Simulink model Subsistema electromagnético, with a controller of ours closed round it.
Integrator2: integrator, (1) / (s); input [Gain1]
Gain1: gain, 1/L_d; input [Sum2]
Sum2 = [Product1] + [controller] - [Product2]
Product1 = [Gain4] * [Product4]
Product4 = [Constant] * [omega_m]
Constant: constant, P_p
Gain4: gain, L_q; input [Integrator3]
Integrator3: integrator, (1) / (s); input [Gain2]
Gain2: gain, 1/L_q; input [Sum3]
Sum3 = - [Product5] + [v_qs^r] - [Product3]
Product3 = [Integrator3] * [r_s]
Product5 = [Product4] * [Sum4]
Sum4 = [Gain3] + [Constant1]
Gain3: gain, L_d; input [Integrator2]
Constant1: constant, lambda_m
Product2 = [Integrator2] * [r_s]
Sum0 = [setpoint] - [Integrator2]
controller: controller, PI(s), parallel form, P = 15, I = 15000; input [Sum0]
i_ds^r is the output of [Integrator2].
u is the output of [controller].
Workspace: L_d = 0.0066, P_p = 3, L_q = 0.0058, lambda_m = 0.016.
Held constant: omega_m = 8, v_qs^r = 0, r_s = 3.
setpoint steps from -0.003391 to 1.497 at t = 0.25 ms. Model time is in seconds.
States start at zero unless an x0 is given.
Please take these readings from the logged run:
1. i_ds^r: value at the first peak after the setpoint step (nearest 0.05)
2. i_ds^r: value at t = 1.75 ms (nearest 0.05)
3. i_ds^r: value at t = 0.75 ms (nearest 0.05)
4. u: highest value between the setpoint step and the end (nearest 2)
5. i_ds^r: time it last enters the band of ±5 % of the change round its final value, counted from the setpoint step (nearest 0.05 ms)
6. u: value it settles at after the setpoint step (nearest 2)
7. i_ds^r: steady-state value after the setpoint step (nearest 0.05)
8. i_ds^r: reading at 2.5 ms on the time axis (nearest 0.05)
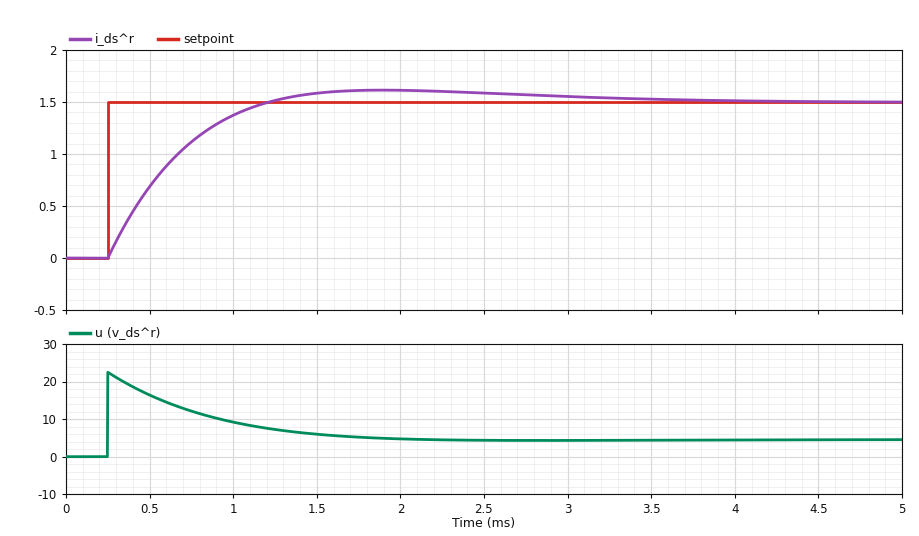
1.60
1.60
1.10
22
2.45 ms
4
1.50
1.60
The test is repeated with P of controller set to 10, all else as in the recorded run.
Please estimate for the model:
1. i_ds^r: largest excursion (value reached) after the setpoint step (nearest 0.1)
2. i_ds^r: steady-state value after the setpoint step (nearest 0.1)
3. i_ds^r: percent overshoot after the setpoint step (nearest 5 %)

1.7
1.5
15 %
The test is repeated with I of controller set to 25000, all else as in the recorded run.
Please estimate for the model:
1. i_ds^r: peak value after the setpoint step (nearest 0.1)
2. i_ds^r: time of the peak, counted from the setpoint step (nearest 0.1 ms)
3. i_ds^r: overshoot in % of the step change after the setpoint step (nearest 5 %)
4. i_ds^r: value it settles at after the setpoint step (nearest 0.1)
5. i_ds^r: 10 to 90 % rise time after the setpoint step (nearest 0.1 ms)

1.7
1.3 ms
15 %
1.5
0.5 ms
